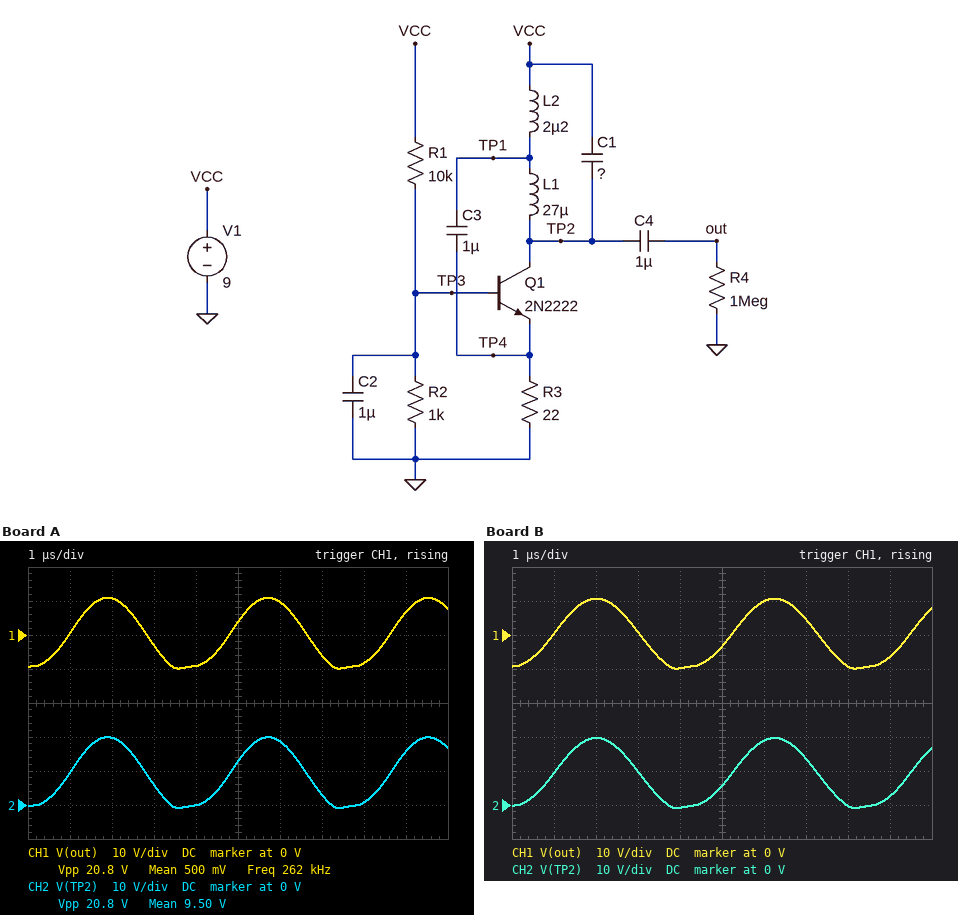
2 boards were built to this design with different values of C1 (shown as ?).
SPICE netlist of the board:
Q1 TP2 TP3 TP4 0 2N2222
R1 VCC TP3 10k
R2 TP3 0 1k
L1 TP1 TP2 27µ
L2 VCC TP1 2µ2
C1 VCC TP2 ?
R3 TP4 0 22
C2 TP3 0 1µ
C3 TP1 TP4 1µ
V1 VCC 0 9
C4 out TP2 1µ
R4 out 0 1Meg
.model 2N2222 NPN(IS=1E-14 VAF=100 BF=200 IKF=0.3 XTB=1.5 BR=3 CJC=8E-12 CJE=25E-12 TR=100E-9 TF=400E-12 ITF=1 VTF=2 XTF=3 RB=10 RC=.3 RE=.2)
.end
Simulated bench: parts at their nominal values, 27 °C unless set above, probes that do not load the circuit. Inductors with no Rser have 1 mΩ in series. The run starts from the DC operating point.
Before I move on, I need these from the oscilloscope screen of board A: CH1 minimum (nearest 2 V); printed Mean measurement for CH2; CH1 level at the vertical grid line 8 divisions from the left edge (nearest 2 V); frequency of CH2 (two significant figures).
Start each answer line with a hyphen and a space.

- -10 V
- 9.50 V
- -8 V
- 260 kHz
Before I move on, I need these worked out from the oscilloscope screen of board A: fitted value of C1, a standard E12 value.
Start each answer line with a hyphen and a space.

- 12 nF
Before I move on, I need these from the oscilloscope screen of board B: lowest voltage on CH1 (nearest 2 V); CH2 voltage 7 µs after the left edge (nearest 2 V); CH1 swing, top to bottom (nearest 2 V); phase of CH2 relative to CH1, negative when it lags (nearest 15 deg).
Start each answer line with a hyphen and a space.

- -10 V
- 14 V
- 20 V
- 0 deg
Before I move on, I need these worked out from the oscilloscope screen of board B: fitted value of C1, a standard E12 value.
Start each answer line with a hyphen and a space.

- 15 nF
